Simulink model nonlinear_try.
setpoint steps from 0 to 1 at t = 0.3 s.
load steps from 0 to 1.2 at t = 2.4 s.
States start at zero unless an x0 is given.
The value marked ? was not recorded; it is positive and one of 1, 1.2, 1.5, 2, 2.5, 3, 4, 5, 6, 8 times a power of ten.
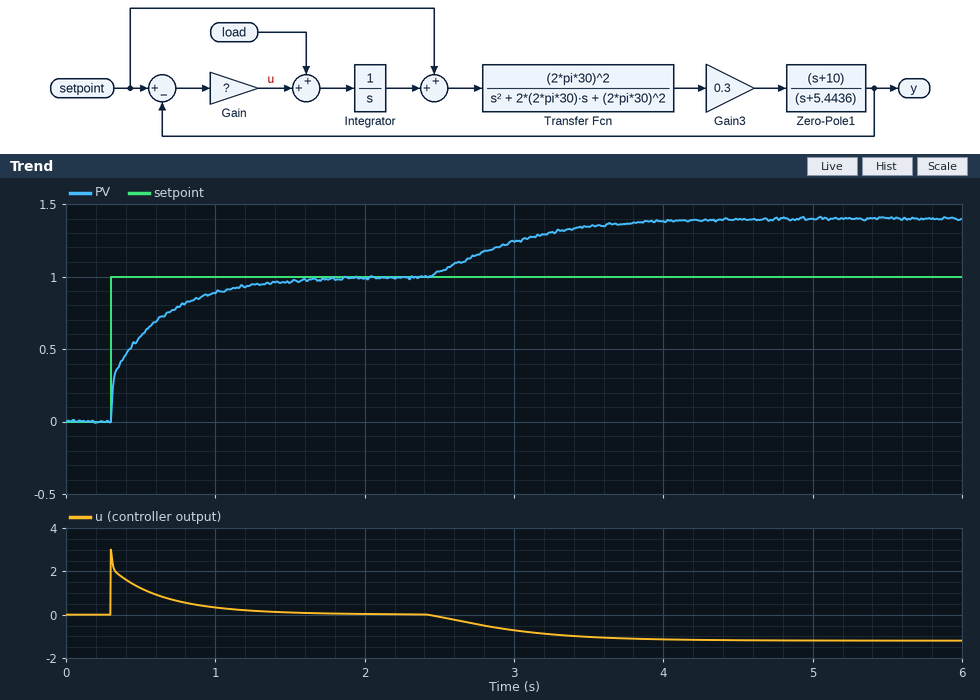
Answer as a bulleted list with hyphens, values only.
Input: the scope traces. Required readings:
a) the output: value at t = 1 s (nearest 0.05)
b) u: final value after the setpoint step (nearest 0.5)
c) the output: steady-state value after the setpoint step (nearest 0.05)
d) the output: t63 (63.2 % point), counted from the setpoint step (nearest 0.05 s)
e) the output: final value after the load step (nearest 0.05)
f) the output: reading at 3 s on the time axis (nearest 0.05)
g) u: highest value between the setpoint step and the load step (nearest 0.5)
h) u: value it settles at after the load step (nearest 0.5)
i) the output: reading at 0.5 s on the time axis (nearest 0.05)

- 0.90
- 0.0
- 1.00
- 0.25 s
- 1.40
- 1.25
- 3.0
- -1.0
- 0.60
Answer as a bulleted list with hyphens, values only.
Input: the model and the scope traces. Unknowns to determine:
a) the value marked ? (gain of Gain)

- 3
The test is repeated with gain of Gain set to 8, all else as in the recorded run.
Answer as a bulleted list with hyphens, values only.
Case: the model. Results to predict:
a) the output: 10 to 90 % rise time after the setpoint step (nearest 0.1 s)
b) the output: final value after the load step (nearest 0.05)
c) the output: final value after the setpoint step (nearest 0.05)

- 0.3 s
- 1.15
- 1.00
